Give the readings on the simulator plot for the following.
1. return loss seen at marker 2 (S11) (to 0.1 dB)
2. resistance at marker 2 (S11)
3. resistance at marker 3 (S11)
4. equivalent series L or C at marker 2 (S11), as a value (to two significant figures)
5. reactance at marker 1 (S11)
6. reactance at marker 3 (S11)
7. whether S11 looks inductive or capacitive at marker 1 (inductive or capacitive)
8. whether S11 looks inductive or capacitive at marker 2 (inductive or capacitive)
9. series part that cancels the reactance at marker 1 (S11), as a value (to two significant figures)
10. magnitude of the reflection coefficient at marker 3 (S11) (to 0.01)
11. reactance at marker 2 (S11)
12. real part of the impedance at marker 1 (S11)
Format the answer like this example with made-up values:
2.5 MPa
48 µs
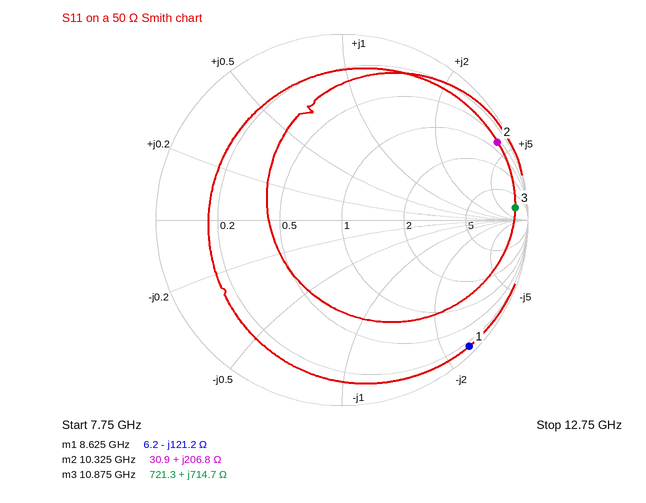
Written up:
0.6 dB
30.9 Ω
721.3 Ω
3.2 nH
-121.2 Ω
+714.7 Ω
capacitive
inductive
2.2 nH
0.93
+206.8 Ω
6.2 Ω
